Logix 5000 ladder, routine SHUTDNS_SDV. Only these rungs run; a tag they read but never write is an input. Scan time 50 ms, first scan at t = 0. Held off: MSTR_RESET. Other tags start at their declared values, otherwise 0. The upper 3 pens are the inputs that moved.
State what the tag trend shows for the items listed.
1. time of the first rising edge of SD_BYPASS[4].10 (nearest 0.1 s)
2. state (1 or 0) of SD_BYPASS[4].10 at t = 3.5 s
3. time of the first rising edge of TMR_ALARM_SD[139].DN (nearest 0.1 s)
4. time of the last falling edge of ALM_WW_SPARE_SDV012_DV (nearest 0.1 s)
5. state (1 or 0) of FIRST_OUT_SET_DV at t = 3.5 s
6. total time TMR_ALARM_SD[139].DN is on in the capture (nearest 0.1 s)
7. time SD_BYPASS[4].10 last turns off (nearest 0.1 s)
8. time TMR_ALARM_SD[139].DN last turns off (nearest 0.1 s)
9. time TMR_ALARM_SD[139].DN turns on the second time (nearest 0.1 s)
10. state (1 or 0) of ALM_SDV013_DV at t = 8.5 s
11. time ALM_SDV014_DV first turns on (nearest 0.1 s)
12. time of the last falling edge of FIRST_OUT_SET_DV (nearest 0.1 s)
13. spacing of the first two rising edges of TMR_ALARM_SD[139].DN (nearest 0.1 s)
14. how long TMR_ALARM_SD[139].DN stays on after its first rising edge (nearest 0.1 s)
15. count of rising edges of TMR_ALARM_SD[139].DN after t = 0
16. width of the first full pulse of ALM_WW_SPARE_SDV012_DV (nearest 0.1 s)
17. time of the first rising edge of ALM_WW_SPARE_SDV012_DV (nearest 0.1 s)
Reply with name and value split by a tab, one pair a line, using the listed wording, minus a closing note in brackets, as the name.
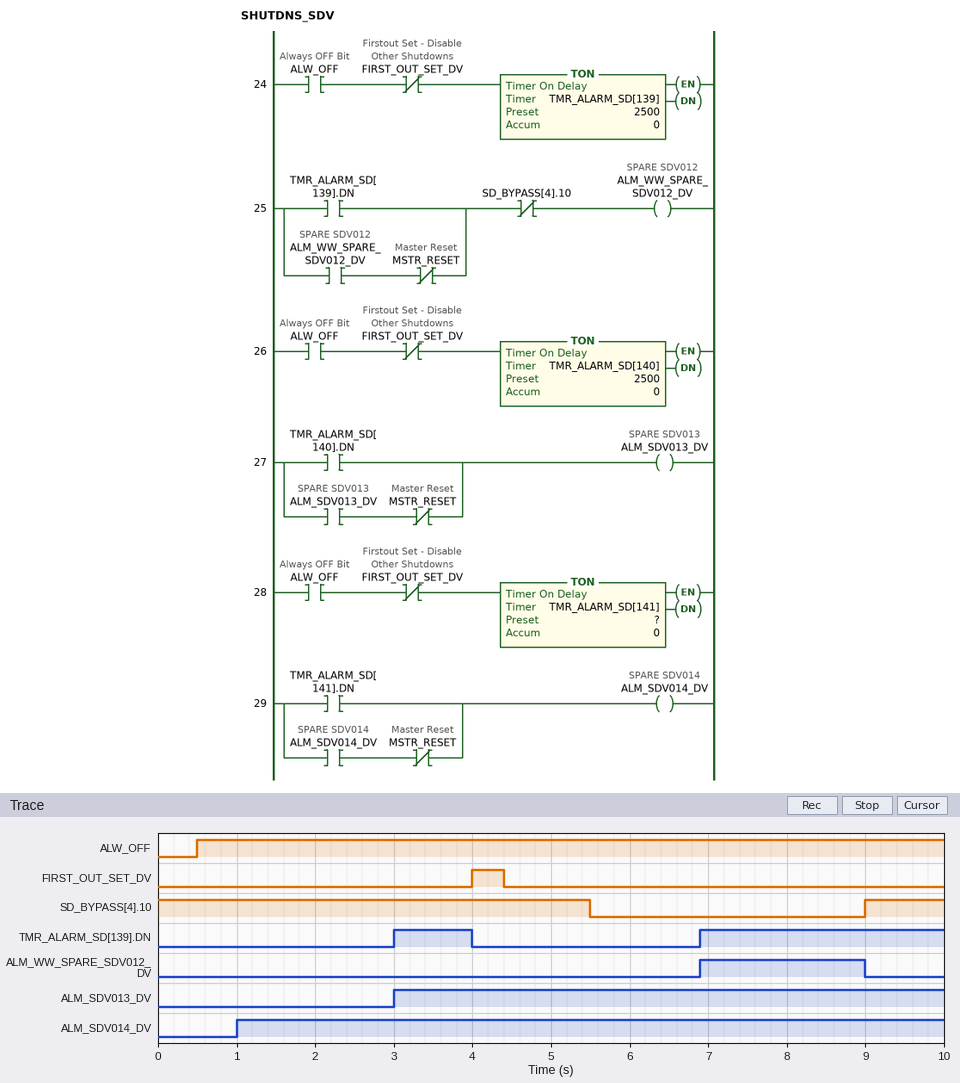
time of the first rising edge of SD_BYPASS[4].10	9.0 s
state (1 or 0) of SD_BYPASS[4].10 at t = 3.5 s	1
time of the first rising edge of TMR_ALARM_SD[139].DN	3.0 s
time of the last falling edge of ALM_WW_SPARE_SDV012_DV	9.0 s
state (1 or 0) of FIRST_OUT_SET_DV at t = 3.5 s	0
total time TMR_ALARM_SD[139].DN is on in the capture	4.1 s
time SD_BYPASS[4].10 last turns off	5.5 s
time TMR_ALARM_SD[139].DN last turns off	4.0 s
time TMR_ALARM_SD[139].DN turns on the second time	6.9 s
state (1 or 0) of ALM_SDV013_DV at t = 8.5 s	1
time ALM_SDV014_DV first turns on	1.0 s
time of the last falling edge of FIRST_OUT_SET_DV	4.4 s
spacing of the first two rising edges of TMR_ALARM_SD[139].DN	3.9 s
how long TMR_ALARM_SD[139].DN stays on after its first rising edge	1.0 s
count of rising edges of TMR_ALARM_SD[139].DN after t = 0	2
width of the first full pulse of ALM_WW_SPARE_SDV012_DV	2.1 s
time of the first rising edge of ALM_WW_SPARE_SDV012_DV	6.9 s
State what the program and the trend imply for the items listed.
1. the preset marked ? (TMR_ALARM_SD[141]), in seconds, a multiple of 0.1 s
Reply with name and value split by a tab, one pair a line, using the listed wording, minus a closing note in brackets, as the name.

the preset marked ? (TMR_ALARM_SD[141]), in seconds, a multiple of 0.1 s	0.5 s
